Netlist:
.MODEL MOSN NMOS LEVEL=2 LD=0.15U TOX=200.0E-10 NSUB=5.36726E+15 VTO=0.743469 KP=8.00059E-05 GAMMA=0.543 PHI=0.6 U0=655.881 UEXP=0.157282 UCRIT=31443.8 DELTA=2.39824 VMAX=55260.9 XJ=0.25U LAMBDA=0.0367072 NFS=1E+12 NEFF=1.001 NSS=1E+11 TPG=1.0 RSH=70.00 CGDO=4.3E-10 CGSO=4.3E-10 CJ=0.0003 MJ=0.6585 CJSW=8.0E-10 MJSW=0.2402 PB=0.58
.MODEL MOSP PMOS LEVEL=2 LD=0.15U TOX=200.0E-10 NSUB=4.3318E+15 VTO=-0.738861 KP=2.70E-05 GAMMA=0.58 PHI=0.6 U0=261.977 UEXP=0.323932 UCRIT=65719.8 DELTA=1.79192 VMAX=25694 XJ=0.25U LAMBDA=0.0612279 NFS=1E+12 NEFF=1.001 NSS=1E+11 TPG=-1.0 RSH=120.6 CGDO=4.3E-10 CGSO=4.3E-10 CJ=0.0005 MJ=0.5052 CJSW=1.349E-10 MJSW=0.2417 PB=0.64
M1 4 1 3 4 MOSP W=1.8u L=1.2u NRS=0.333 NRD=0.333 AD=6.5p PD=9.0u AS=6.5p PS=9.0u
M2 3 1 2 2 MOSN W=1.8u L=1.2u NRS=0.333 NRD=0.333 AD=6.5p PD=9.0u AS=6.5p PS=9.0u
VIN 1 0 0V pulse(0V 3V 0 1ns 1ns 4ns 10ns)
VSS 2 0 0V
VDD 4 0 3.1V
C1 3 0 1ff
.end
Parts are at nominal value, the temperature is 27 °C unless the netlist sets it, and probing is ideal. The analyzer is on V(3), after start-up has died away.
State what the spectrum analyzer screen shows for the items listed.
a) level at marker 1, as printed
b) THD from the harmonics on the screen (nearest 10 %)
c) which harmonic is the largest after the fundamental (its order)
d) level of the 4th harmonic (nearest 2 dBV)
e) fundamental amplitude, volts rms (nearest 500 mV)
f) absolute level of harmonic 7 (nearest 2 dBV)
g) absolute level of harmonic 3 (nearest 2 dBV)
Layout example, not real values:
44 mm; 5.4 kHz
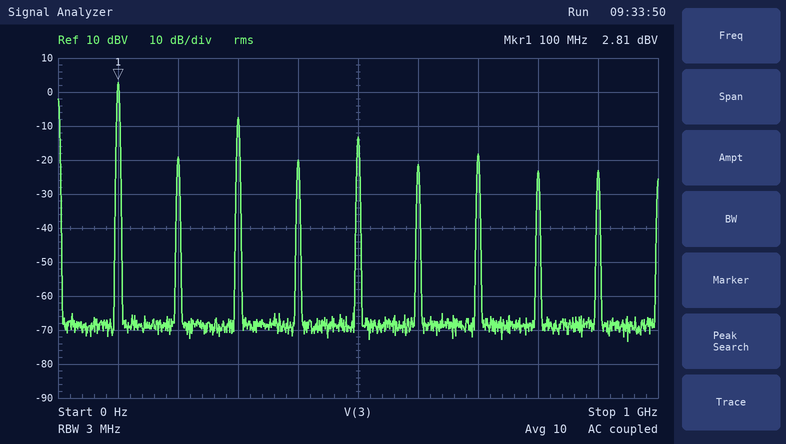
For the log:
2.81 dBV; 40 %; 3; -20 dBV; 1.5 V; -18 dBV; -8 dBV
